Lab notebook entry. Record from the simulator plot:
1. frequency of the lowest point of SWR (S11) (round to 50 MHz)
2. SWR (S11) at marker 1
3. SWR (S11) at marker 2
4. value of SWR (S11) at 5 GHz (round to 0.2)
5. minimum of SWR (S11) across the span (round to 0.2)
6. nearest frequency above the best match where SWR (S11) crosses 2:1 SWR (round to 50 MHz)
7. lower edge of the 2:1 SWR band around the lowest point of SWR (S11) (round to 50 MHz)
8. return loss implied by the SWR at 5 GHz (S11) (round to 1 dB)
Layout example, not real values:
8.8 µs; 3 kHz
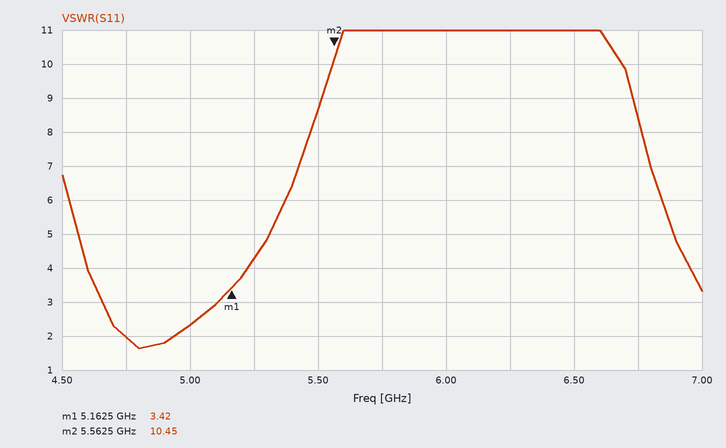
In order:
4.80 GHz; 3.42; 10.45; 2.4; 1.6; 4.95 GHz; 4.75 GHz; 8 dB
